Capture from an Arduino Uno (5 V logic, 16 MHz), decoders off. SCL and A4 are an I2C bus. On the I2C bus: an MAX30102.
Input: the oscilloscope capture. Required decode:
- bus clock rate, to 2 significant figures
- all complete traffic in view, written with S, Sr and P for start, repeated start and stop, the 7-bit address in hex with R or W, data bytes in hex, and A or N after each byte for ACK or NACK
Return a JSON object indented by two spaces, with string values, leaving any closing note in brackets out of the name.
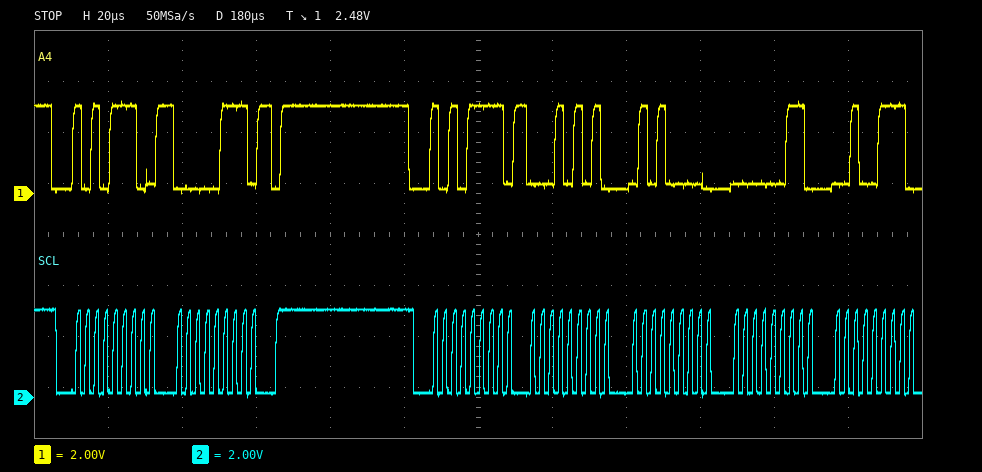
{
  "bus clock rate, to 2 significant figures": "400 kHz",
  "all complete traffic in view, written with S, Sr and P for start, repeated start and stop, the 7-bit address in hex with R or W, data bytes in hex, and A or N after each byte for ACK or NACK": "S 57W A 07 A P S 57R A 15 A 50 A 03 A 27 A"
}
